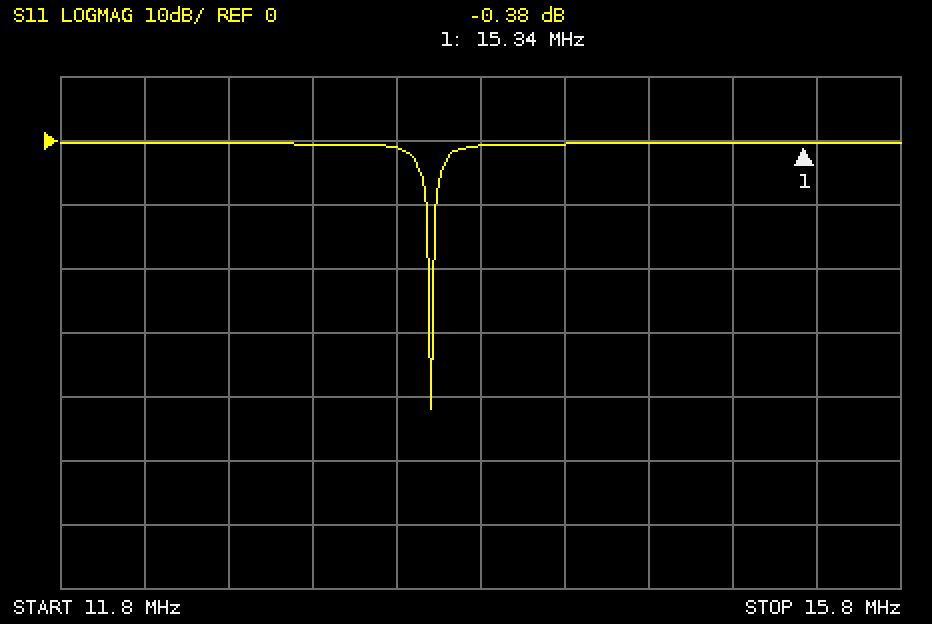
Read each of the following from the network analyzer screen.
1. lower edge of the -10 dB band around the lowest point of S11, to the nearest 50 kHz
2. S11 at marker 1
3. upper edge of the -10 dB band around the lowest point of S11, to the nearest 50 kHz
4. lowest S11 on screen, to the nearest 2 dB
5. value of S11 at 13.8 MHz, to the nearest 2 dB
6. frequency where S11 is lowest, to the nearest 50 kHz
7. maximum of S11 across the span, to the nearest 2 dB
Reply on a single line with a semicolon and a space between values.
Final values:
13.55 MHz; -0.38 dB; 13.60 MHz; -42 dB; 0 dB; 13.55 MHz; 0 dB
